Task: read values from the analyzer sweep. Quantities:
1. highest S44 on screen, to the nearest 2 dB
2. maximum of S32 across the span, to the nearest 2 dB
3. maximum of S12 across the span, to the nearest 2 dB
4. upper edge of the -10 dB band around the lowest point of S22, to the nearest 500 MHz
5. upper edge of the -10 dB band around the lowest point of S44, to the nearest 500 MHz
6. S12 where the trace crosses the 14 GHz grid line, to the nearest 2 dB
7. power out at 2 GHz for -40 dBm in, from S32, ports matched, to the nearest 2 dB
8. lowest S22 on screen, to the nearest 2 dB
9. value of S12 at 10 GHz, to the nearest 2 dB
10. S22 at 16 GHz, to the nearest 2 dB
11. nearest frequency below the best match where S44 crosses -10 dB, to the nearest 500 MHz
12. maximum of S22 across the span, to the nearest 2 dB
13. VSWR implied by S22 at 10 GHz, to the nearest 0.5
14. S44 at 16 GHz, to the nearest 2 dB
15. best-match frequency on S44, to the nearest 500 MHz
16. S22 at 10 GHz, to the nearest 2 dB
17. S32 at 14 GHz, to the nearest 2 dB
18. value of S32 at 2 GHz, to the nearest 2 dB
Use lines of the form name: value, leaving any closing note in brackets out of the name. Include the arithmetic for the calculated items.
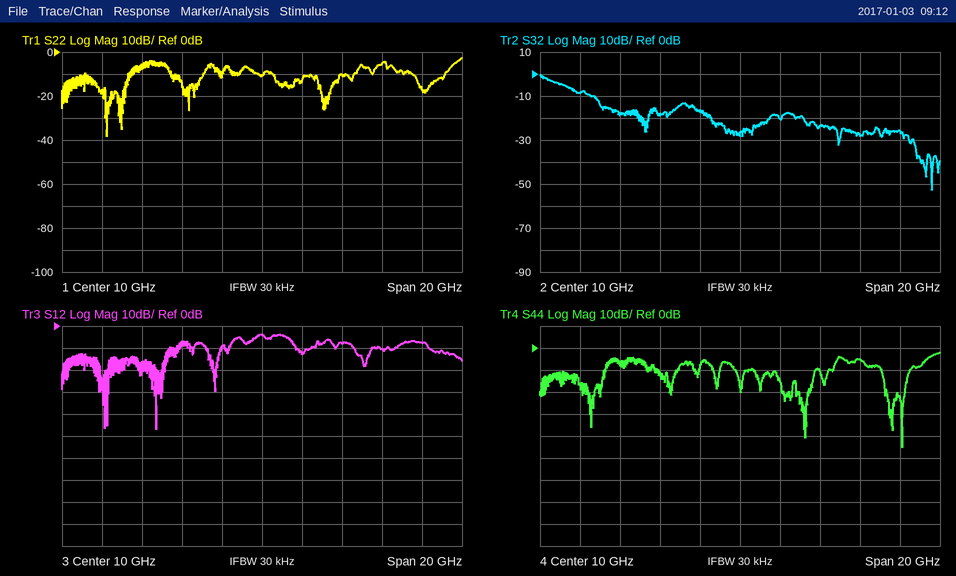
highest S44 on screen, to the nearest 2 dB: -2 dB
maximum of S32 across the span, to the nearest 2 dB: 0 dB
maximum of S12 across the span, to the nearest 2 dB: -4 dB
upper edge of the -10 dB band around the lowest point of S22, to the nearest 500 MHz: 3.5 GHz
upper edge of the -10 dB band around the lowest point of S44, to the nearest 500 MHz: 18.5 GHz
S12 where the trace crosses the 14 GHz grid line, to the nearest 2 dB: -8 dB
power out at 2 GHz for -40 dBm in, from S32, ports matched, to the nearest 2 dB: -40 dBm + (-8 dB) = -48 dBm
lowest S22 on screen, to the nearest 2 dB: -38 dB
value of S12 at 10 GHz, to the nearest 2 dB: -4 dB
S22 at 16 GHz, to the nearest 2 dB: -6 dB
nearest frequency below the best match where S44 crosses -10 dB, to the nearest 500 MHz: 17.0 GHz
maximum of S22 across the span, to the nearest 2 dB: -2 dB
VSWR implied by S22 at 10 GHz, to the nearest 0.5: |Γ| = 10^(-10/20) = 0.3162; VSWR = (1 + 0.3162)/(1 − 0.3162) ≈ 1.92, so 2.0 to the nearest 0.5
S44 at 16 GHz, to the nearest 2 dB: -6 dB
best-match frequency on S44, to the nearest 500 MHz: 18.0 GHz
S22 at 10 GHz, to the nearest 2 dB: -10 dB
S32 at 14 GHz, to the nearest 2 dB: -24 dB
value of S32 at 2 GHz, to the nearest 2 dB: -8 dB
